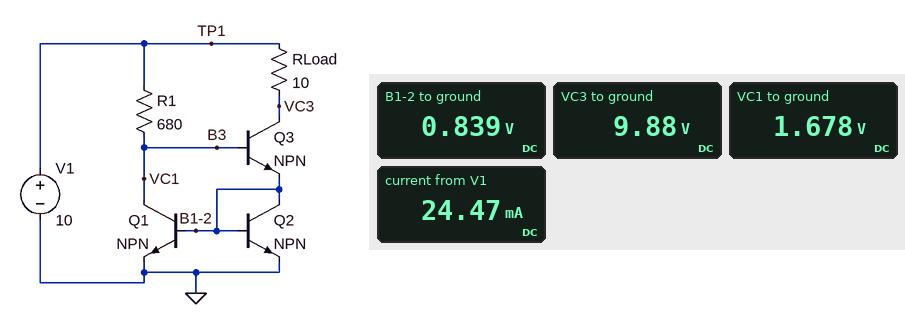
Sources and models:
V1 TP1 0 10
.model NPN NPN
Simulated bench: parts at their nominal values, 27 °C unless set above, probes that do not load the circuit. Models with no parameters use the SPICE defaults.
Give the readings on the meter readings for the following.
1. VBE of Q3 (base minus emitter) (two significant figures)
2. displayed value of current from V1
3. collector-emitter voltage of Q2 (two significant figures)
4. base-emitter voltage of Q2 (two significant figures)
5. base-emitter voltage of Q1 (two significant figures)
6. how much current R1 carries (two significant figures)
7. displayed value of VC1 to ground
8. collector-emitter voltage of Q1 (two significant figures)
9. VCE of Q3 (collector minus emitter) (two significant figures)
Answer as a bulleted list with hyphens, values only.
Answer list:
- 840 mV
- 24.47 mA
- 840 mV
- 840 mV
- 840 mV
- 12 mA
- 1.678 V
- 1.7 V
- 9.0 V
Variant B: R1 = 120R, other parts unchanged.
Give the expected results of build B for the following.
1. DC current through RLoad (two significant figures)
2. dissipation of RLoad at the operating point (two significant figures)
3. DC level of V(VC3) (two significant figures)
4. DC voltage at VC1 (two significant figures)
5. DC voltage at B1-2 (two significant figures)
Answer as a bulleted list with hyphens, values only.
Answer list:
- 69 mA
- 47 mW
- 9.3 V
- 1.8 V
- 880 mV
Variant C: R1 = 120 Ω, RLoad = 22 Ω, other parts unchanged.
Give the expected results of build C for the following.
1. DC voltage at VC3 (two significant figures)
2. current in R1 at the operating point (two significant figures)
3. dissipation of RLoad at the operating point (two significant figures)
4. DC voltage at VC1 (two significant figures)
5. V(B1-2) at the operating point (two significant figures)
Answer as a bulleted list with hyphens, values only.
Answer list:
- 8.5 V
- 69 mA
- 100 mW
- 1.8 V
- 880 mV
